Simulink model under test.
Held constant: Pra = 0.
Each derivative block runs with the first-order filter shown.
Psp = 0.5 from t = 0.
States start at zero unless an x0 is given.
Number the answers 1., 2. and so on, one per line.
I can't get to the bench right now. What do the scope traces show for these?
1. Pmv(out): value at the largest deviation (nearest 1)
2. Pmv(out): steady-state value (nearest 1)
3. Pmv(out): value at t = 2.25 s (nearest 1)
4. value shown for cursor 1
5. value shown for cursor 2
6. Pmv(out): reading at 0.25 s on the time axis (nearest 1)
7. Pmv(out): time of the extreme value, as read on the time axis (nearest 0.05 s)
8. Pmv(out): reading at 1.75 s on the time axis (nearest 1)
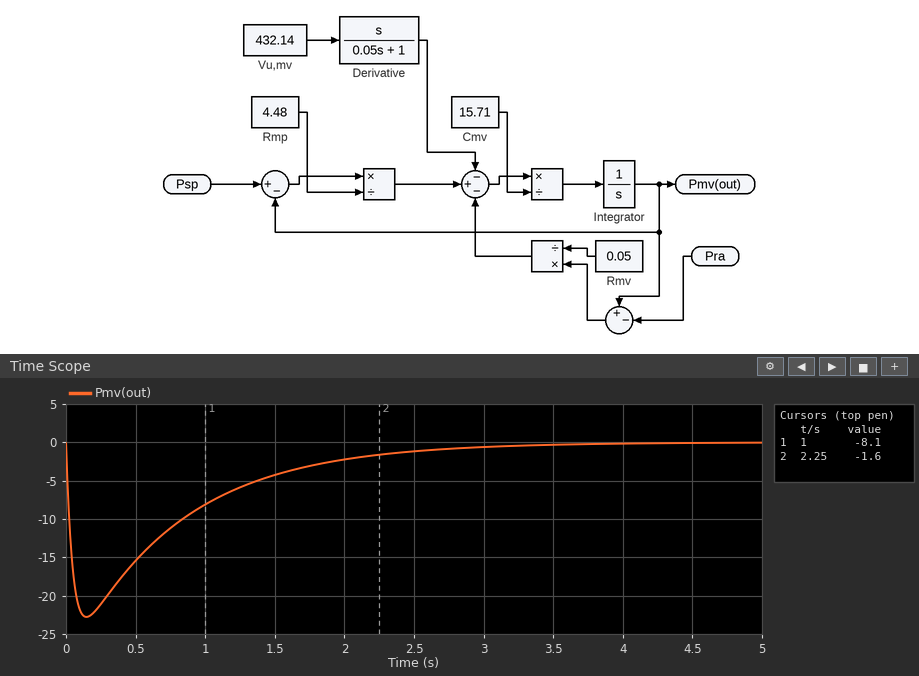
1. -23
2. 0
3. -2
4. -8.1
5. -1.6
6. -21
7. 0.15 s
8. -3
